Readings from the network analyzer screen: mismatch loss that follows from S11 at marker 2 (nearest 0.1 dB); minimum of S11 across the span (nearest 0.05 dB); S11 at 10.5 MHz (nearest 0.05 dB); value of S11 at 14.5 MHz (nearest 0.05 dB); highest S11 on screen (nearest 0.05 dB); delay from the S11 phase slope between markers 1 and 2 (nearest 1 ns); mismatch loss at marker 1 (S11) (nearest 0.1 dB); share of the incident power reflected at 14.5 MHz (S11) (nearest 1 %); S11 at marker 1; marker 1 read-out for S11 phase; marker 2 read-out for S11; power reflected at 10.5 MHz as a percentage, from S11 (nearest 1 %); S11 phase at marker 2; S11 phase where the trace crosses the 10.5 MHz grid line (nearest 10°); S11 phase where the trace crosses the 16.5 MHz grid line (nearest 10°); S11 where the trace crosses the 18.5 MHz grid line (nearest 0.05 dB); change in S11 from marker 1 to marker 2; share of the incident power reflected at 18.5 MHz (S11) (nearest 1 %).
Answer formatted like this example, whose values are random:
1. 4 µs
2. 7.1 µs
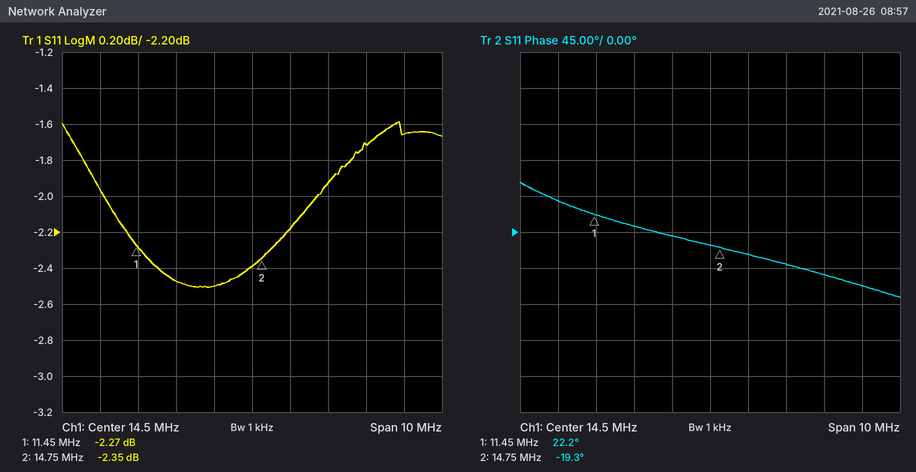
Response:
1. 3.8 dB
2. -2.50 dB
3. -1.95 dB
4. -2.40 dB
5. -1.60 dB
6. 35 ns
7. 3.9 dB
8. 58 %
9. -2.27 dB
10. 22.2°
11. -2.35 dB
12. 64 %
13. -19.3°
14. 40°
15. -40°
16. -1.65 dB
17. -0.08 dB
18. 68 %
